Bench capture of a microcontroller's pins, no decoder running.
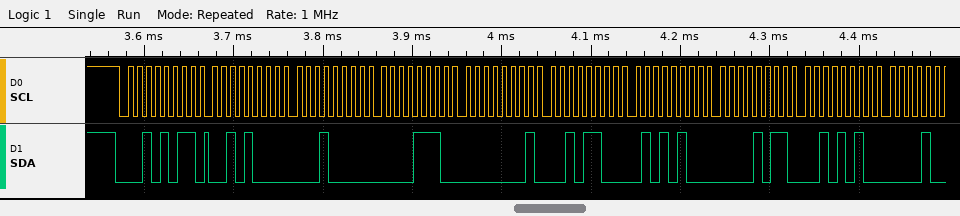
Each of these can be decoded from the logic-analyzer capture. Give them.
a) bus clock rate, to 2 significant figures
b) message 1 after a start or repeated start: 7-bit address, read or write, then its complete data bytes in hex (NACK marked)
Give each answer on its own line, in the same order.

100 kHz
0x15 read: 28 10 0E 01 2C 54 0B 2A
